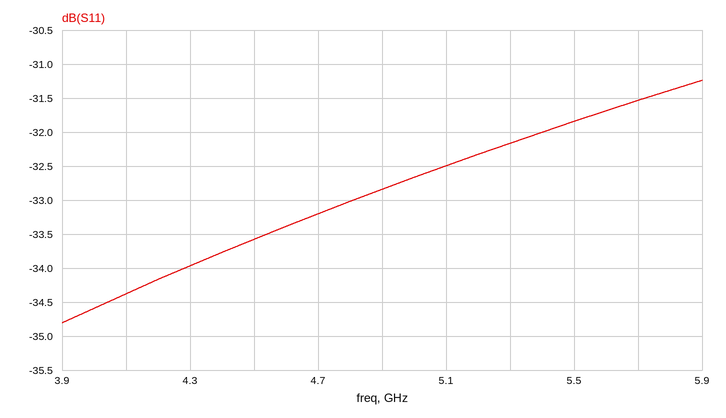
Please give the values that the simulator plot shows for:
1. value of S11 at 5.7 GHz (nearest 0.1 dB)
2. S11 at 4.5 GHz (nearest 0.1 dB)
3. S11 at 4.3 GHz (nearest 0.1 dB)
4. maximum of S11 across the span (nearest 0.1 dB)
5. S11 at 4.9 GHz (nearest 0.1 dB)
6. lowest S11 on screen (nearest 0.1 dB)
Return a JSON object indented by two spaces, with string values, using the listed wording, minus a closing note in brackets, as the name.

{
  "value of S11 at 5.7 GHz": "-31.5 dB",
  "S11 at 4.5 GHz": "-33.6 dB",
  "S11 at 4.3 GHz": "-34.0 dB",
  "maximum of S11 across the span": "-31.2 dB",
  "S11 at 4.9 GHz": "-32.8 dB",
  "lowest S11 on screen": "-34.8 dB"
}
